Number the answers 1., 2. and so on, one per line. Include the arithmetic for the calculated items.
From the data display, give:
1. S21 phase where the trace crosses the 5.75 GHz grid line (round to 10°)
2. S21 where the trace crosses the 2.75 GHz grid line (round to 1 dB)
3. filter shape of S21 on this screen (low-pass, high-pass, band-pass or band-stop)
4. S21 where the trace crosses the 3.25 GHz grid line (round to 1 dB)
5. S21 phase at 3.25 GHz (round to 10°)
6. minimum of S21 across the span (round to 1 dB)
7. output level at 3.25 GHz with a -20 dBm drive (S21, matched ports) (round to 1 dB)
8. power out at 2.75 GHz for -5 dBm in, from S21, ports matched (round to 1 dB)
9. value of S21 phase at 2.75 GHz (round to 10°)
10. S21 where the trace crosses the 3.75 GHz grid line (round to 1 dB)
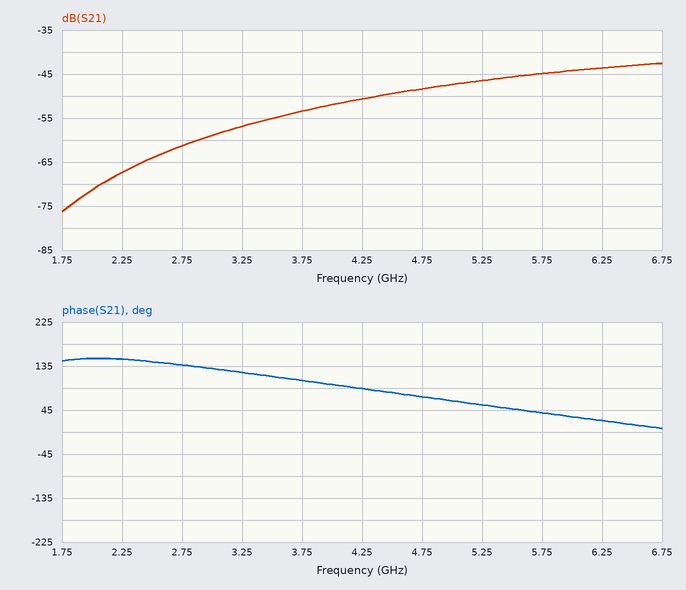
1. 40°
2. -61 dB
3. high-pass
4. -57 dB
5. 120°
6. -76 dB
7. -20 dBm + (-57 dB) = -77 dBm
8. -5 dBm + (-61 dB) = -66 dBm
9. 140°
10. -53 dB
